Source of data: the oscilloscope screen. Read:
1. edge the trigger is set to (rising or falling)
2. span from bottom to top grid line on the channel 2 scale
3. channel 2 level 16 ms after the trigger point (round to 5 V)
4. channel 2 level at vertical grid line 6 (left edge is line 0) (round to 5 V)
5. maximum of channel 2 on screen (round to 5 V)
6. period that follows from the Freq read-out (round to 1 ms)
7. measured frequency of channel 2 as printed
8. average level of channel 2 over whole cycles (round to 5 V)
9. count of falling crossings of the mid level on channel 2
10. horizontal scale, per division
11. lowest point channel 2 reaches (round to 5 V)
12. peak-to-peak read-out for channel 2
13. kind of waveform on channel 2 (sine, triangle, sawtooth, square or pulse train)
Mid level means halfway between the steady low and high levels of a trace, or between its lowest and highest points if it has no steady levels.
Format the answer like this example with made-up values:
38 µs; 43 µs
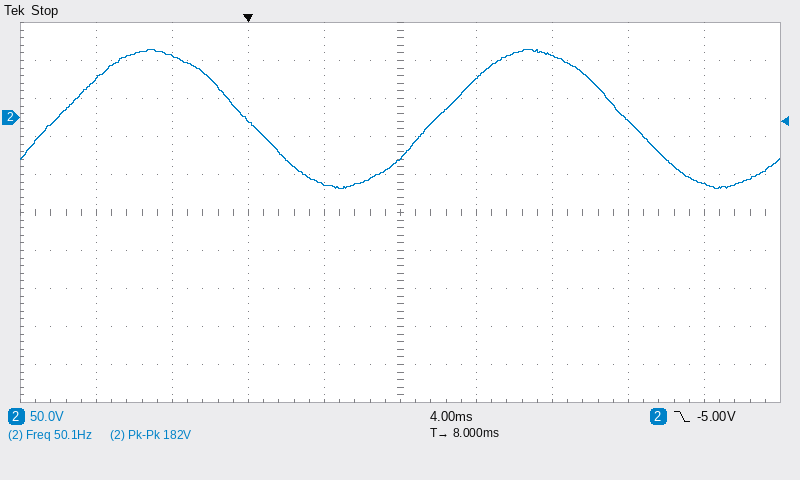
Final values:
falling; 500 V; 80 V; 50 V; 90 V; 20 ms; 50.1 Hz; 0 V; 2; 4 ms; -95 V; 182 V; sine
